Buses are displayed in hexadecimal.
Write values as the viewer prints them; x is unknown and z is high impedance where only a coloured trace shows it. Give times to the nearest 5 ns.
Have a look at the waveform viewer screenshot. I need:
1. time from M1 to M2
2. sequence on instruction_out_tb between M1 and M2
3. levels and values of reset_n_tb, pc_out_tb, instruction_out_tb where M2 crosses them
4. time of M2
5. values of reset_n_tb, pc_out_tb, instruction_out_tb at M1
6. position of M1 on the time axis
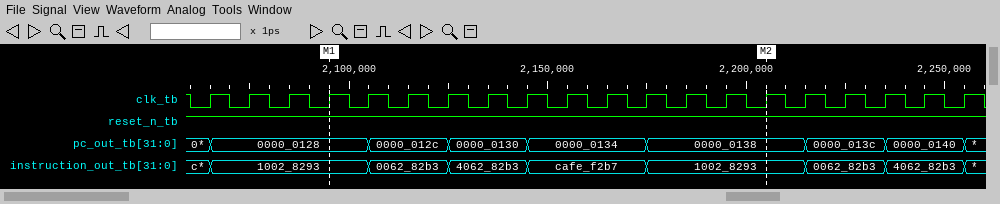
110 ns
1002_8293, 0062_82b3, 4062_82b3, cafe_f2b7, 1002_8293
reset_n_tb=1, pc_out_tb=0000_0138, instruction_out_tb=1002_8293
2205 ns
reset_n_tb=1, pc_out_tb=0000_0128, instruction_out_tb=1002_8293
2095 ns
